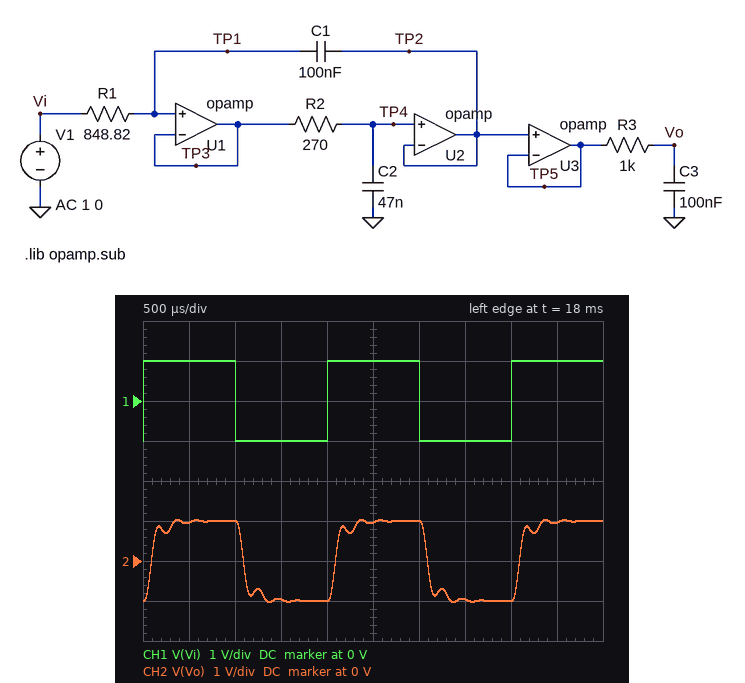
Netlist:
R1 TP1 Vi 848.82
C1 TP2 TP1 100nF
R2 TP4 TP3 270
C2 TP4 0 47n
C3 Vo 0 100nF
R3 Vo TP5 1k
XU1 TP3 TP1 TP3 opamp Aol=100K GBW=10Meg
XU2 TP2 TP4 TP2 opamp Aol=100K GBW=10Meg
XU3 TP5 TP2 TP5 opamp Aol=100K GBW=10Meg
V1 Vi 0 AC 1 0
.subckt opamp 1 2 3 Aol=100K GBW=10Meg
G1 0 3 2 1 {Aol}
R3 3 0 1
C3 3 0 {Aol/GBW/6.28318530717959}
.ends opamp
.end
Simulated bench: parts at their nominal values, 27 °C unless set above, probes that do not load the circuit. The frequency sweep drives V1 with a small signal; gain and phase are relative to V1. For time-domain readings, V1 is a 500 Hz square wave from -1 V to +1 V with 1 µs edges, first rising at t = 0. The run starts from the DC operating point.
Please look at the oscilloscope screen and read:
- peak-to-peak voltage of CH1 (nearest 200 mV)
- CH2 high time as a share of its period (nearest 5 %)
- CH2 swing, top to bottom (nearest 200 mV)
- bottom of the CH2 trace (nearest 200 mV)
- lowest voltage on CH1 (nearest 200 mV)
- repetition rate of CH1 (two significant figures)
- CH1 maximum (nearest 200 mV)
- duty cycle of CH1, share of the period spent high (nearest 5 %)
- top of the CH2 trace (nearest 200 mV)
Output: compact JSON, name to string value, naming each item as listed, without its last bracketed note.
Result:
{"peak-to-peak voltage of CH1": "2.0 V", "CH2 high time as a share of its period": "50 %", "CH2 swing, top to bottom": "2.0 V", "bottom of the CH2 trace": "-1.0 V", "lowest voltage on CH1": "-1.0 V", "repetition rate of CH1": "500 Hz", "CH1 maximum": "1.0 V", "duty cycle of CH1, share of the period spent high": "50 %", "top of the CH2 trace": "1.0 V"}
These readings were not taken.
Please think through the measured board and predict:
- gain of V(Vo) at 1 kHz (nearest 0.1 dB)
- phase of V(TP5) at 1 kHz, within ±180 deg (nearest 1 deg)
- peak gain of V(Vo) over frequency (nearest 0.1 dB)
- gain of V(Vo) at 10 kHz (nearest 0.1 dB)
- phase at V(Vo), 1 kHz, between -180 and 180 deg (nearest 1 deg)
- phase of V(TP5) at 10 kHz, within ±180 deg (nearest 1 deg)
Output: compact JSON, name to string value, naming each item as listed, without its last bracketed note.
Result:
{"gain of V(Vo) at 1 kHz": "-1.1 dB", "phase of V(TP5) at 1 kHz, within ±180 deg": "-5 deg", "peak gain of V(Vo) over frequency": "0 dB", "gain of V(Vo) at 10 kHz": "-26.6 dB", "phase at V(Vo), 1 kHz, between -180 and 180 deg": "-37 deg", "phase of V(TP5) at 10 kHz, within ±180 deg": "-166 deg"}
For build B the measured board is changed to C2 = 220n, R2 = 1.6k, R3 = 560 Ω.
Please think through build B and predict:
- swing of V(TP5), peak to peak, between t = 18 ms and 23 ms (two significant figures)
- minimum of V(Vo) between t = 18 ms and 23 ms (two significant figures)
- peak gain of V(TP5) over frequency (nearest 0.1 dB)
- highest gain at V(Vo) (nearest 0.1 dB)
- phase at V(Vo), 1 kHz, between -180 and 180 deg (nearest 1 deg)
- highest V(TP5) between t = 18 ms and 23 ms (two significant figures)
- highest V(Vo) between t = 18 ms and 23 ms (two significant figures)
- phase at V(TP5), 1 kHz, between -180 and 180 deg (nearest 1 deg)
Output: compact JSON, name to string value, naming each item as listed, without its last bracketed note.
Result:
{"swing of V(TP5), peak to peak, between t = 18 ms and 23 ms": "1.9 V", "minimum of V(Vo) between t = 18 ms and 23 ms": "-940 mV", "peak gain of V(TP5) over frequency": "0 dB", "highest gain at V(Vo)": "0 dB", "phase at V(Vo), 1 kHz, between -180 and 180 deg": "-114 deg", "highest V(TP5) between t = 18 ms and 23 ms": "950 mV", "highest V(Vo) between t = 18 ms and 23 ms": "940 mV", "phase at V(TP5), 1 kHz, between -180 and 180 deg": "-95 deg"}
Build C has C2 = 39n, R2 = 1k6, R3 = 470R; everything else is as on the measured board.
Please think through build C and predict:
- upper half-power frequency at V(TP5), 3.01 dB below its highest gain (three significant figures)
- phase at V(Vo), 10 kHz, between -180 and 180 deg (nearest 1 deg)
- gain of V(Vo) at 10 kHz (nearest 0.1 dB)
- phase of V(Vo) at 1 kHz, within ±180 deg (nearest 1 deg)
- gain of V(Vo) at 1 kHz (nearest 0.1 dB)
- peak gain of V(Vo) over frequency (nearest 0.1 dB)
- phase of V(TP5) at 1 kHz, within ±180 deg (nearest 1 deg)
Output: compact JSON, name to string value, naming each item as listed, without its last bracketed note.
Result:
{"upper half-power frequency at V(TP5), 3.01 dB below its highest gain": "2.59 kHz", "phase at V(Vo), 10 kHz, between -180 and 180 deg": "120 deg", "gain of V(Vo) at 10 kHz": "-36.0 dB", "phase of V(Vo) at 1 kHz, within ±180 deg": "-43 deg", "gain of V(Vo) at 1 kHz": "0.7 dB", "peak gain of V(Vo) over frequency": "1.3 dB", "phase of V(TP5) at 1 kHz, within ±180 deg": "-26 deg"}
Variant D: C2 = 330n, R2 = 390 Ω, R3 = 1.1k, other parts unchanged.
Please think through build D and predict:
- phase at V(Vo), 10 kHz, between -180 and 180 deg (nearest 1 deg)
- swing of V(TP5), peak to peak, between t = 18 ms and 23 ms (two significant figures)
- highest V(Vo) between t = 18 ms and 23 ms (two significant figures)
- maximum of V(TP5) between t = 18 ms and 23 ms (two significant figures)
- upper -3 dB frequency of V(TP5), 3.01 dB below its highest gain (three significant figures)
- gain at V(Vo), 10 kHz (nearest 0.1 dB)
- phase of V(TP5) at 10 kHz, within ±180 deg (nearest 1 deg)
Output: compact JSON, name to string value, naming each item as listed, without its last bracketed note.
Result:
{"phase at V(Vo), 10 kHz, between -180 and 180 deg": "109 deg", "swing of V(TP5), peak to peak, between t = 18 ms and 23 ms": "2.3 V", "highest V(Vo) between t = 18 ms and 23 ms": "1.1 V", "maximum of V(TP5) between t = 18 ms and 23 ms": "1.2 V", "upper -3 dB frequency of V(TP5), 3.01 dB below its highest gain": "1.68 kHz", "gain at V(Vo), 10 kHz": "-49.5 dB", "phase of V(TP5) at 10 kHz, within ±180 deg": "-169 deg"}
